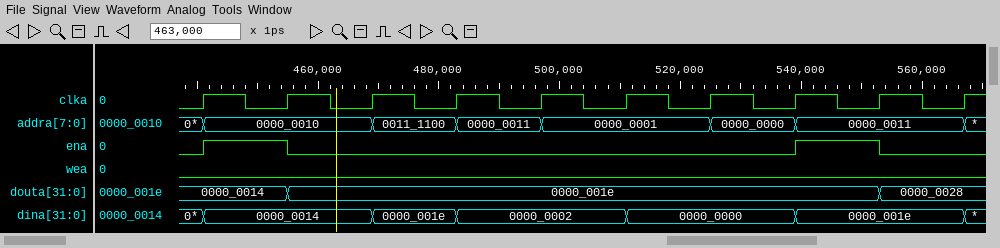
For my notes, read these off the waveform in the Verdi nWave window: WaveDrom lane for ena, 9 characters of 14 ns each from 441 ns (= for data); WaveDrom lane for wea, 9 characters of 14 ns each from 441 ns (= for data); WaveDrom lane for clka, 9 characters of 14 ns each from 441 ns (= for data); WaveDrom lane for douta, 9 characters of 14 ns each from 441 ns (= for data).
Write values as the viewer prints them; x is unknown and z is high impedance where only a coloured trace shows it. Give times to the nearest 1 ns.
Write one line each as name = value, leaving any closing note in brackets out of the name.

WaveDrom lane for ena, 9 characters of 14 ns each from 441 ns = {name: 'ena', wave: '10.....10'}
WaveDrom lane for wea, 9 characters of 14 ns each from 441 ns = {name: 'wea', wave: '0........'}
WaveDrom lane for clka, 9 characters of 14 ns each from 441 ns = {name: 'clka', wave: 'p........'}
WaveDrom lane for douta, 9 characters of 14 ns each from 441 ns = {name: 'douta', wave: '==......=', data: '0000_0014 0000_001e 0000_0028'}
